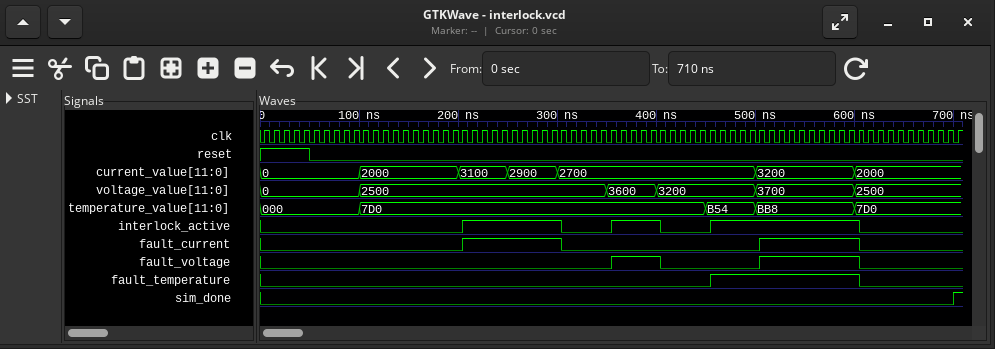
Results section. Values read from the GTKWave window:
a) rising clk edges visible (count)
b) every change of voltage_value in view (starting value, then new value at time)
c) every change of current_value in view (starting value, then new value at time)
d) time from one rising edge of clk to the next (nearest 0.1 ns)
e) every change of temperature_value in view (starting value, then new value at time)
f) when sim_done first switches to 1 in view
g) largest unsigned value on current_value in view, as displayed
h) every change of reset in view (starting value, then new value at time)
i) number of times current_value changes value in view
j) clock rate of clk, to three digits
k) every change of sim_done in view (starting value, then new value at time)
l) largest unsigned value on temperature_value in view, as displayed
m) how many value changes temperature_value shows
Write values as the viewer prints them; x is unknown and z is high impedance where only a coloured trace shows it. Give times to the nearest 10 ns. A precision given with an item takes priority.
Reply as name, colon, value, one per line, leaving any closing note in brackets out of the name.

rising clk edges visible: 71
every change of voltage_value in view: 0, 2500 at 100 ns, 3600 at 350 ns, 3200 at 400 ns, 3700 at 500 ns, 2500 at 600 ns
every change of current_value in view: 0, 2000 at 100 ns, 3100 at 200 ns, 2900 at 250 ns, 2700 at 300 ns, 3200 at 500 ns, 2000 at 600 ns
time from one rising edge of clk to the next: 10 ns
every change of temperature_value in view: 000, 7D0 at 100 ns, B54 at 450 ns, BB8 at 500 ns, 7D0 at 600 ns
when sim_done first switches to 1 in view: 700 ns
largest unsigned value on current_value in view, as displayed: 3200
every change of reset in view: 1, 0 at 50 ns
number of times current_value changes value in view: 6
clock rate of clk, to three digits: 100 MHz
every change of sim_done in view: 0, 1 at 700 ns
largest unsigned value on temperature_value in view, as displayed: BB8
how many value changes temperature_value shows: 4
